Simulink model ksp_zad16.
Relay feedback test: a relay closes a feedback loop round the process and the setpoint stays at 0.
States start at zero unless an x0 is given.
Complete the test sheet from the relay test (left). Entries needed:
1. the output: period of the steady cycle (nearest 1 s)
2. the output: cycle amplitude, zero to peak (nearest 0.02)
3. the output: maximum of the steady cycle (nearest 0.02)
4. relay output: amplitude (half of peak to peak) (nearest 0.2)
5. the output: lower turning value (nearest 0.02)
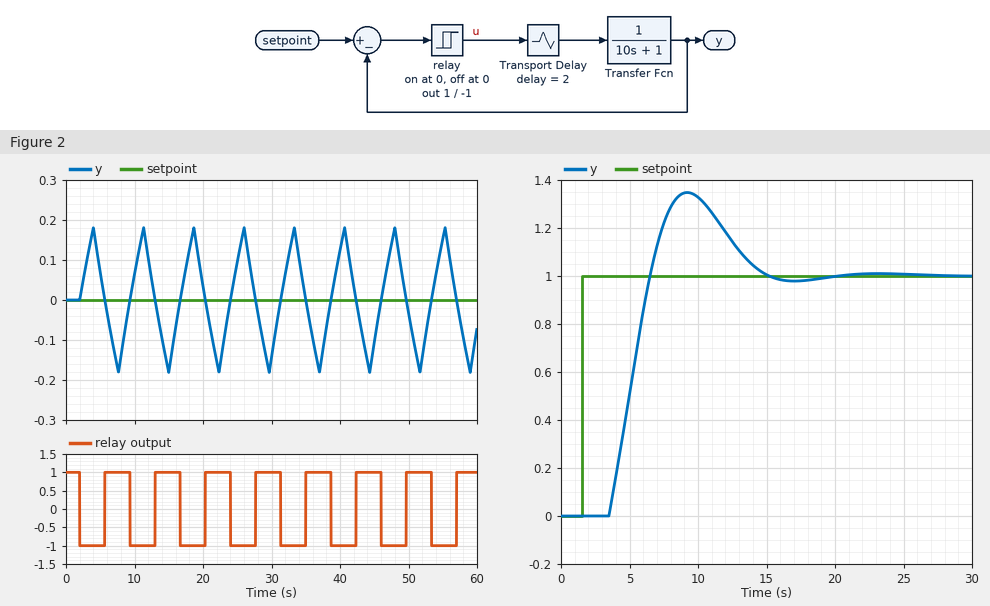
7 s
0.18
0.18
1.0
-0.18
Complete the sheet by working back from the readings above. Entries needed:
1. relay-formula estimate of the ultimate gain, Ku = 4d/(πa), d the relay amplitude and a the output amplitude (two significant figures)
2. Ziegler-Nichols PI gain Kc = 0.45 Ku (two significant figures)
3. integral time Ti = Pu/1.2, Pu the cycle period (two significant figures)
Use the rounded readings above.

7.1
3.2
5.8 s
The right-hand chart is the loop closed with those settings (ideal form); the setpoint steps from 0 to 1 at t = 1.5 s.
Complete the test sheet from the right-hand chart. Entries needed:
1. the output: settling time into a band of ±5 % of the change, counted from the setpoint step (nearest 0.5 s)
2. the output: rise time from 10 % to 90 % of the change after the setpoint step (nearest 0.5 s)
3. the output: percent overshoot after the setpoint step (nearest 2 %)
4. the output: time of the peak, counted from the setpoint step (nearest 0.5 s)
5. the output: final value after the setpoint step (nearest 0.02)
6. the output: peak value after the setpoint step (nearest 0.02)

12.5 s
2.5 s
34 %
7.5 s
1.00
1.34
